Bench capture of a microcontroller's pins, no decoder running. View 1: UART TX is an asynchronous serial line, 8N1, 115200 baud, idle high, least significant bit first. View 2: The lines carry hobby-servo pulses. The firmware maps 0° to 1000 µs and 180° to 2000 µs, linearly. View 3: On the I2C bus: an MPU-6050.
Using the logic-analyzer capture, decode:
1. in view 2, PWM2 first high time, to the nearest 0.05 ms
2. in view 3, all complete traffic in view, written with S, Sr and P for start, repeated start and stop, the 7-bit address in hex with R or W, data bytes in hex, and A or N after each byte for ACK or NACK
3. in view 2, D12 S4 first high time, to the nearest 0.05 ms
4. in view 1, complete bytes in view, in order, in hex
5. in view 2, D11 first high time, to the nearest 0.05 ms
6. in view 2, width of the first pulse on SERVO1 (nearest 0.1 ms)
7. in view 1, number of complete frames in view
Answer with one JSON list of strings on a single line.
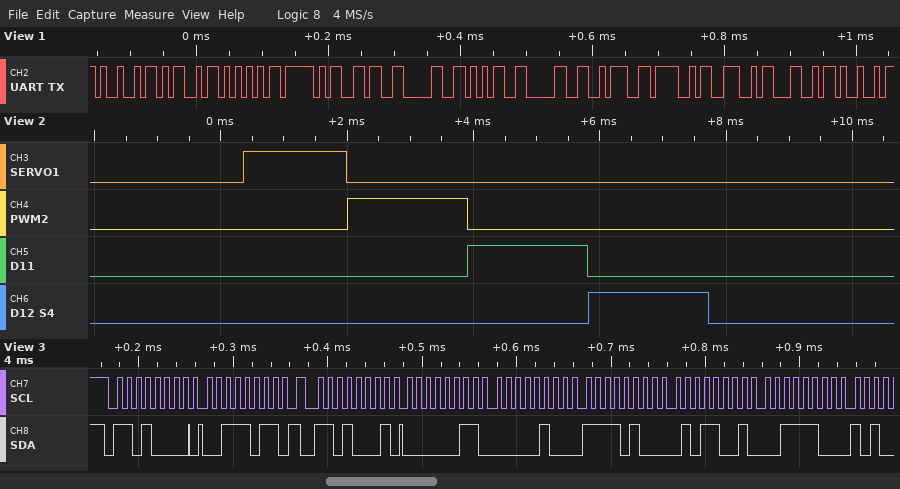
["1.90 ms", "S 68W A 3B A Sr 68R A 03 A 04 A F4 A 59 A 3C A", "1.90 ms", "49 4D 55 5F 36 30 35 30 3A 4F 4E 4C 49", "1.90 ms", "1.6 ms", "13"]
